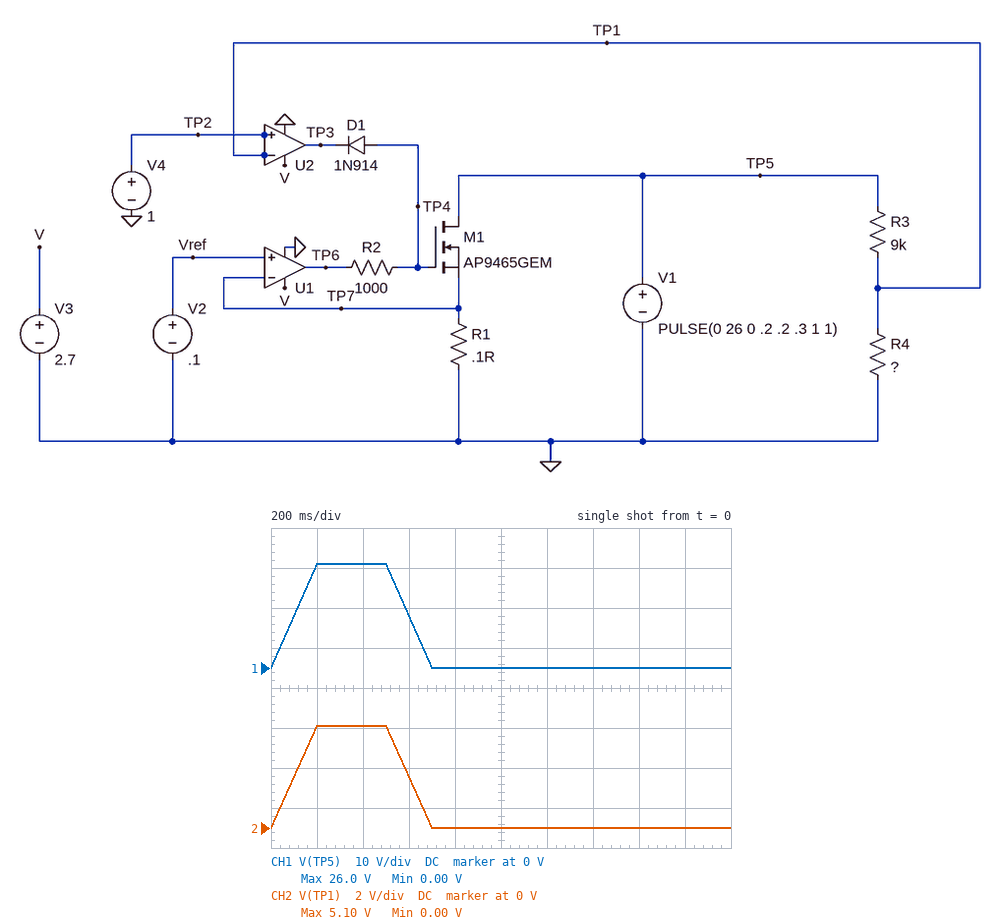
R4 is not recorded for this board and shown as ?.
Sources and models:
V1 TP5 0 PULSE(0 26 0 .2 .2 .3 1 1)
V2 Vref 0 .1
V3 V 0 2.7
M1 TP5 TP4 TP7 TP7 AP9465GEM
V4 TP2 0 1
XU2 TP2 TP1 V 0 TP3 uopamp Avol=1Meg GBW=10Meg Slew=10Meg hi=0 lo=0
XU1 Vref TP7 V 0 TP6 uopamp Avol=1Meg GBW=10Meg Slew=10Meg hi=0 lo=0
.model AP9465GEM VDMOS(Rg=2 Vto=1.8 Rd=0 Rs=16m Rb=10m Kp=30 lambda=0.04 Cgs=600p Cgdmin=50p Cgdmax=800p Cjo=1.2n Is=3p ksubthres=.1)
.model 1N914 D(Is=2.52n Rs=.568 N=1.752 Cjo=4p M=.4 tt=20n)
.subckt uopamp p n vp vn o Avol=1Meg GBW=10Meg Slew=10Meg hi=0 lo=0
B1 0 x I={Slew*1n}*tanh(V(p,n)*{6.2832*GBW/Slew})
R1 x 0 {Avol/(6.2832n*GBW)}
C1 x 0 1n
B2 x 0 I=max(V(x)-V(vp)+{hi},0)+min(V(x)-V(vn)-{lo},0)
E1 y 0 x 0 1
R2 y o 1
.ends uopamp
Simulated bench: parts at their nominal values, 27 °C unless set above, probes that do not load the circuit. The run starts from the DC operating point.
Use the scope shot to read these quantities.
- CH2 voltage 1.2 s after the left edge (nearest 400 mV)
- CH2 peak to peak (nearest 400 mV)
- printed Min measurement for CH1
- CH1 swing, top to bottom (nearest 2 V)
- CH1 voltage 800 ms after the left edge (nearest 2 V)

0 V
5.2 V
0.00 V
26 V
0 V
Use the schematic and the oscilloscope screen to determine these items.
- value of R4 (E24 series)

2.2 kΩ
